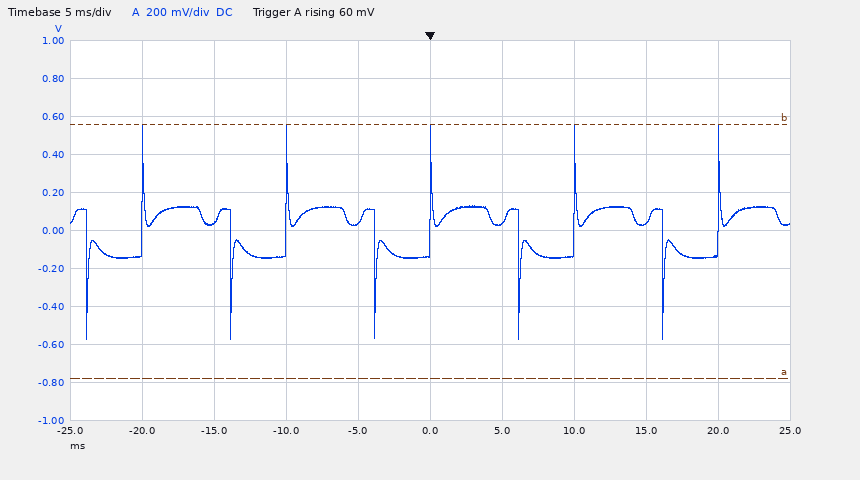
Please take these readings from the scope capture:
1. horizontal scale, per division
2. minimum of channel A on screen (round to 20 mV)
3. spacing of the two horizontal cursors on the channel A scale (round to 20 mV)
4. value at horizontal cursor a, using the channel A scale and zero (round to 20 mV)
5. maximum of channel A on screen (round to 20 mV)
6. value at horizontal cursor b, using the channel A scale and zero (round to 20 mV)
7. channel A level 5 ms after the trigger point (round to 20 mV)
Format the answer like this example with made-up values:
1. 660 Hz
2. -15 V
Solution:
1. 5 ms
2. -580 mV
3. 1.34 V
4. -780 mV
5. 560 mV
6. 560 mV
7. 40 mV
